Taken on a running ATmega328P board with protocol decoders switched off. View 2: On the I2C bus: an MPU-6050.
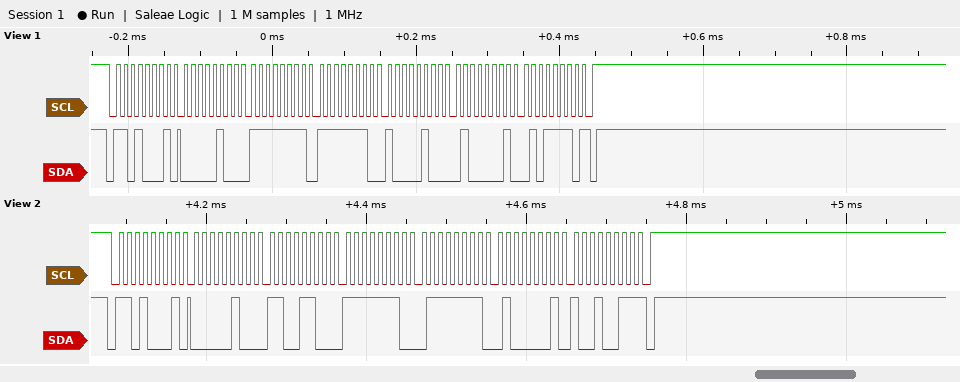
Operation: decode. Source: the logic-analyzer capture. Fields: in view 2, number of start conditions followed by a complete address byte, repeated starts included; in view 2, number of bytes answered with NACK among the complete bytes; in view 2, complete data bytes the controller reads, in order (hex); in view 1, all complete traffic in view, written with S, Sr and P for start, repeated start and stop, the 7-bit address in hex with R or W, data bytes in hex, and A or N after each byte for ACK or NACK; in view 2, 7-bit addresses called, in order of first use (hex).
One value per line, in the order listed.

1
1
04 CC FE 7F 41 93
S 68R A 04 A FF A FE A 84 A 41 A 5E N P
0x68
